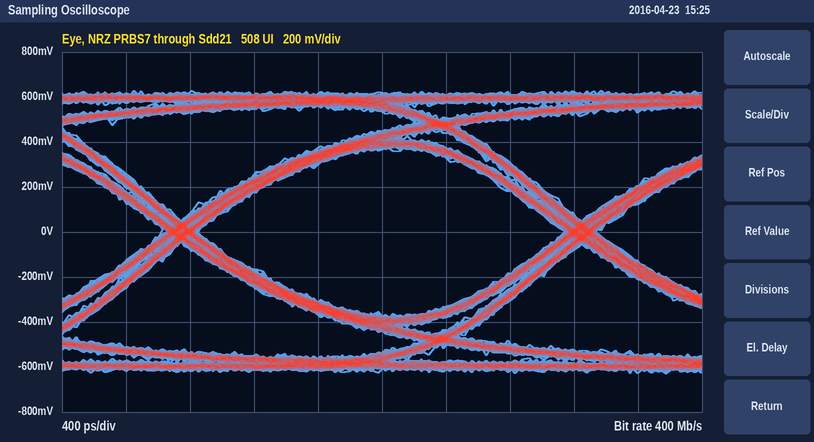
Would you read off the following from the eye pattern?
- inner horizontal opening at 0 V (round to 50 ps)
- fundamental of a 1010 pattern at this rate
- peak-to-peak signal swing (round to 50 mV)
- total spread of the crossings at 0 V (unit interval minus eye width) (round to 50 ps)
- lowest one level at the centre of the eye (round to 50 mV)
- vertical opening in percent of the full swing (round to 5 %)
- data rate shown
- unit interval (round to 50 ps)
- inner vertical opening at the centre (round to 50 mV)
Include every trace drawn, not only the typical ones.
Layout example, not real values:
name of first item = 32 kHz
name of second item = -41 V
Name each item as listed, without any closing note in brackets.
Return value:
inner horizontal opening at 0 V = 2.30 ns
fundamental of a 1010 pattern at this rate = 200 MHz
peak-to-peak signal swing = 1.25 V
total spread of the crossings at 0 V (unit interval minus eye width) = 200 ps
lowest one level at the centre of the eye = 350 mV
vertical opening in percent of the full swing = 60 %
data rate shown = 400 Mb/s
unit interval = 2.50 ns
inner vertical opening at the centre = 750 mV
